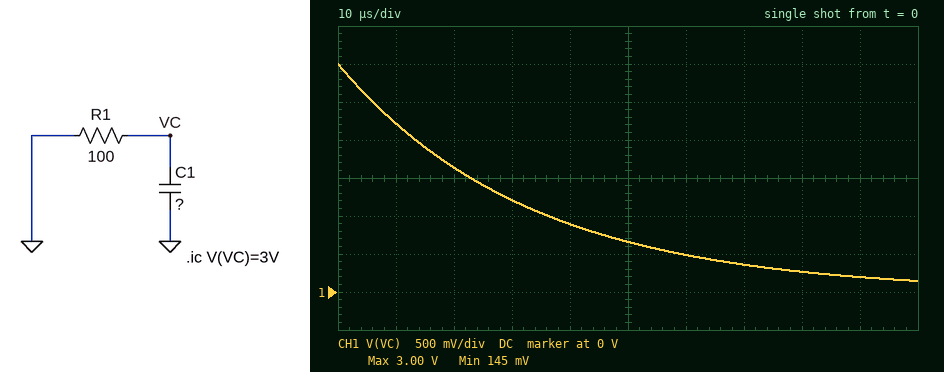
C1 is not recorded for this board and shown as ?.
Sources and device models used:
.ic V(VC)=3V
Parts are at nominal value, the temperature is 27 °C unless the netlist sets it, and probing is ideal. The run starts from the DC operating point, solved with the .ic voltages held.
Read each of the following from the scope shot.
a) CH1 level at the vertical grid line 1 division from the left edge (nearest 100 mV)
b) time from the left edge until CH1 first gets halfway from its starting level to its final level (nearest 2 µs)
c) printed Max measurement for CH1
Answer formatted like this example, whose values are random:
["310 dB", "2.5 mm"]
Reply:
["2.2 V", "22 µs", "3.00 V"]
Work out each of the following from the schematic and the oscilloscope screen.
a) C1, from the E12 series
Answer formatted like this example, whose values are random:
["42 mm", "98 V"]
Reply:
["330 nF"]
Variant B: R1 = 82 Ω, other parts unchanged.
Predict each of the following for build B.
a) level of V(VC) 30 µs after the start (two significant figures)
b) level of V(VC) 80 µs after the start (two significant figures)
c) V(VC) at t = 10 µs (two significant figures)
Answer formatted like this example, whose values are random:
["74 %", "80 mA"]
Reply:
["990 mV", "160 mV", "2.1 V"]
